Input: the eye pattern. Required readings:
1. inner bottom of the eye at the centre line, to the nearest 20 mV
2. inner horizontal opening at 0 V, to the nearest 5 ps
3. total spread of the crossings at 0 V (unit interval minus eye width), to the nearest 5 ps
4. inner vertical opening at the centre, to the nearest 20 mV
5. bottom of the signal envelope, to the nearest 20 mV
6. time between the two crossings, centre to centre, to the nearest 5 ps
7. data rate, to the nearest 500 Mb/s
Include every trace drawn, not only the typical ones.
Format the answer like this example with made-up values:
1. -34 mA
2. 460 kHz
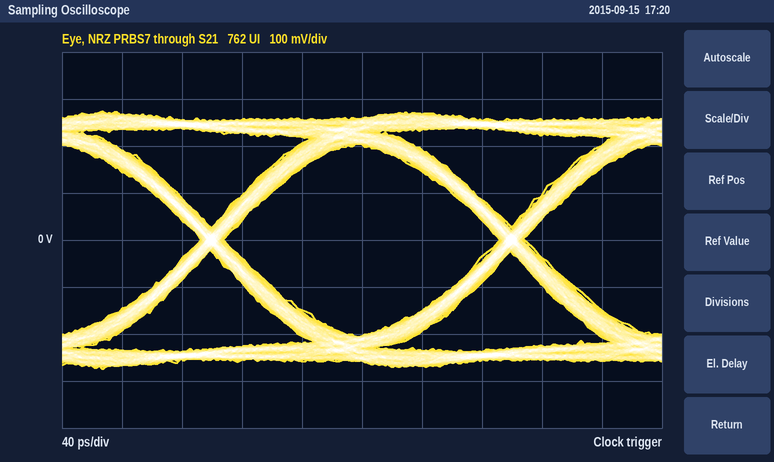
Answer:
1. -200 mV
2. 185 ps
3. 15 ps
4. 400 mV
5. -280 mV
6. 200 ps
7. 5.0 Gb/s
